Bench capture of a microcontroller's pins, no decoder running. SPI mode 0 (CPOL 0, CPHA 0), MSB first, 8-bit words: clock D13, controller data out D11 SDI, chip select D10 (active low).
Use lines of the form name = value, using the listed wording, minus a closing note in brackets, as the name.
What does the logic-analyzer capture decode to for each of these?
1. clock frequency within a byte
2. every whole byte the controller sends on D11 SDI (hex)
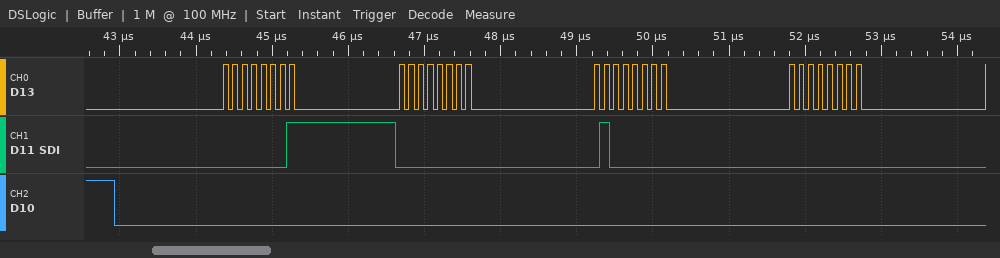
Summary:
clock frequency within a byte = 8 MHz
every whole byte the controller sends on D11 SDI = 01 00 40 00
